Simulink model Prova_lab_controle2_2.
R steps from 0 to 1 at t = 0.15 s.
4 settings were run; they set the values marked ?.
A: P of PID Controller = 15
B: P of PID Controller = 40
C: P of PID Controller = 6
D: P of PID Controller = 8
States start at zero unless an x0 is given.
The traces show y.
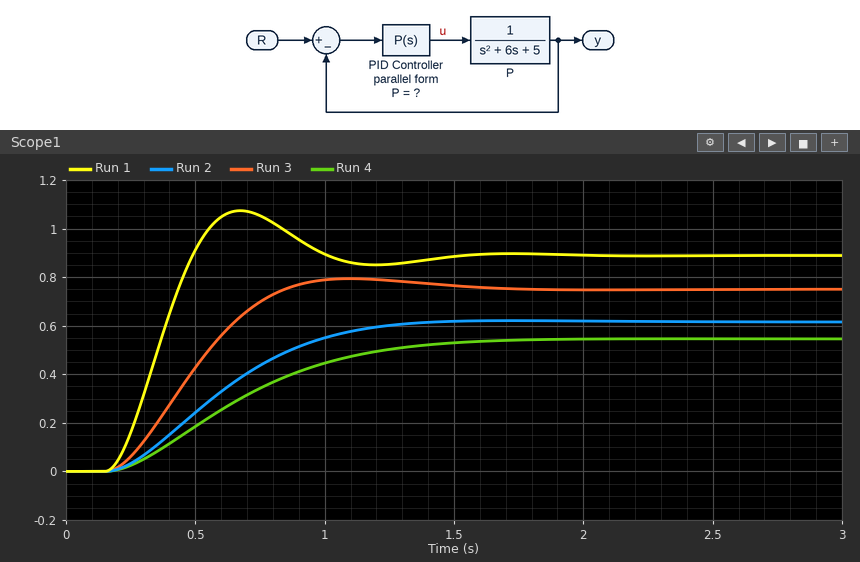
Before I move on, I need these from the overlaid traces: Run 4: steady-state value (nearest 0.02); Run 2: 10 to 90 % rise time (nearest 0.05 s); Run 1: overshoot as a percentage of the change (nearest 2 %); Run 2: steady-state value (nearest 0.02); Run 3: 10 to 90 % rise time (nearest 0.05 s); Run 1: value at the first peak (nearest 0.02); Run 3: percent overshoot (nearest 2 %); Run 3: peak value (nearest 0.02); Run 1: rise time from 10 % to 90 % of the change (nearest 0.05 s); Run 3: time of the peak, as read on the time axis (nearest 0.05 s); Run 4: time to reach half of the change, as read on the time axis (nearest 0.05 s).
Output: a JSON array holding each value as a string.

["0.54", "0.70 s", "20 %", "0.62", "0.45 s", "1.08", "6 %", "0.80", "0.25 s", "1.10 s", "0.65 s"]
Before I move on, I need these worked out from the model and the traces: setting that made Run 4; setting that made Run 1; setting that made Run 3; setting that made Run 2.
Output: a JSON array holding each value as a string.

["C", "B", "A", "D"]
